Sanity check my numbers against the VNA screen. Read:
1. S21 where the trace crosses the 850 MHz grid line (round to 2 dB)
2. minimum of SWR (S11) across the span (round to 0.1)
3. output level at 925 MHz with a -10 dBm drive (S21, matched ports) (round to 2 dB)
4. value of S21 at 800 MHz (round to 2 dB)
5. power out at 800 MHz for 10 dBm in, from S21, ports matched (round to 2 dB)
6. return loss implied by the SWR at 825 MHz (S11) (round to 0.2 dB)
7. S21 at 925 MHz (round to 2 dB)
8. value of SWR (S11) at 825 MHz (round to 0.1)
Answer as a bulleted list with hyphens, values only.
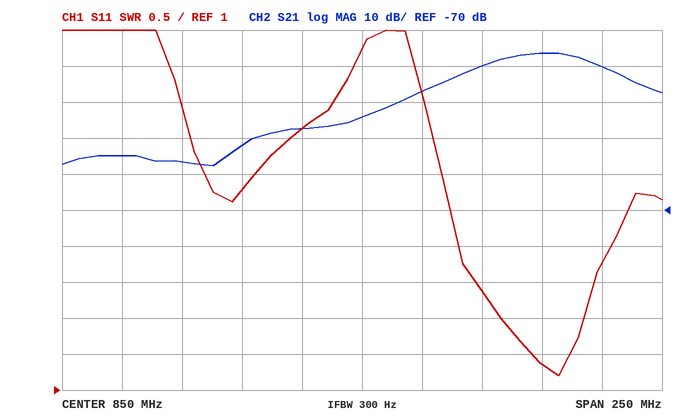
- -44 dB
- 1.2
- -36 dBm
- -52 dB
- -42 dBm
- 3.8 dB
- -26 dB
- 4.6
